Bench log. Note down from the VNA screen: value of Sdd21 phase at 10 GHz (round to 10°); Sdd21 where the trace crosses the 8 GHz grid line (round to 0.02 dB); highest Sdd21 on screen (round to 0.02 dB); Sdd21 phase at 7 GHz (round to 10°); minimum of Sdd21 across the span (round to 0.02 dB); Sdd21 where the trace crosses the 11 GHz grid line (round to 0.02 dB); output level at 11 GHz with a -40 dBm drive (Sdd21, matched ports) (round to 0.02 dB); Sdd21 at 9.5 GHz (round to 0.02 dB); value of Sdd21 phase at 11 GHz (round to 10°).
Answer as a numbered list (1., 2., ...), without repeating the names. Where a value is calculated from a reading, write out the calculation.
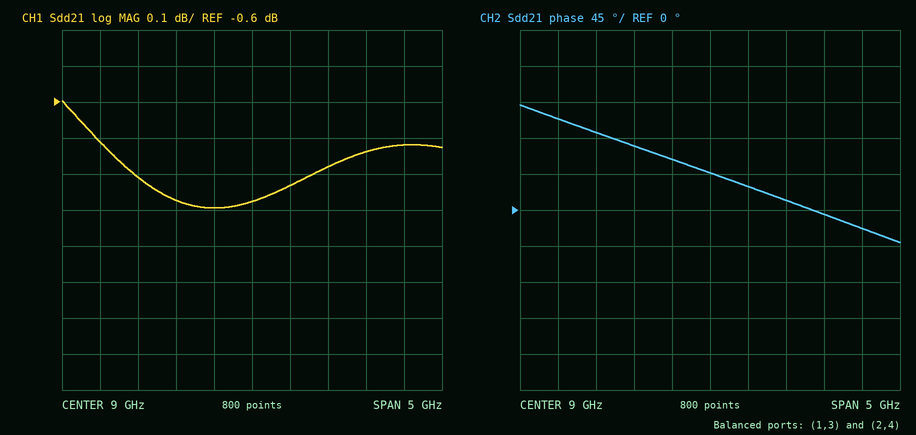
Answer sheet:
1. 10°
2. -0.88 dB
3. -0.60 dB
4. 110°
5. -0.90 dB
6. -0.72 dB
7. -40 dBm + (-0.72 dB) = -40.72 dBm
8. -0.84 dB
9. -20°
